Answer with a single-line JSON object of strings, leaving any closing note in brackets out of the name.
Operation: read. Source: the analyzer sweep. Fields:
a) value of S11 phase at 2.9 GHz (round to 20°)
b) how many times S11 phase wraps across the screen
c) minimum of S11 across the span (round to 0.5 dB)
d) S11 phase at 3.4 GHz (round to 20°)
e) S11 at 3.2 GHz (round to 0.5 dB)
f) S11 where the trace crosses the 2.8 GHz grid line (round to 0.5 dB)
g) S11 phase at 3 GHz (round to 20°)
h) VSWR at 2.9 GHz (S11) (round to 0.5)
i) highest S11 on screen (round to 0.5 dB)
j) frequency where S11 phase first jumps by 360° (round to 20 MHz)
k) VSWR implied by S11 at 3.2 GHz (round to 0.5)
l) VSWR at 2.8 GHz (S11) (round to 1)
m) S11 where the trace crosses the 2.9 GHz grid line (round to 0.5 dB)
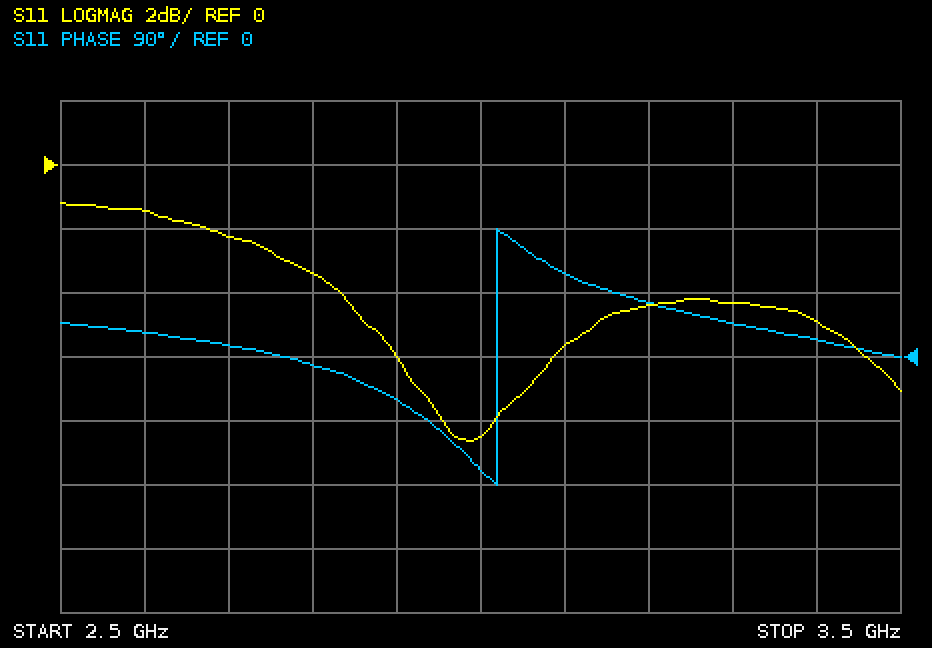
{"value of S11 phase at 2.9 GHz": "-60°", "how many times S11 phase wraps across the screen": "1", "minimum of S11 across the span": "-8.5 dB", "S11 phase at 3.4 GHz": "20°", "S11 at 3.2 GHz": "-4.5 dB", "S11 where the trace crosses the 2.8 GHz grid line": "-3.5 dB", "S11 phase at 3 GHz": "-160°", "VSWR at 2.9 GHz (S11)": "3.0", "highest S11 on screen": "-1.0 dB", "frequency where S11 phase first jumps by 360°": "3.02 GHz", "VSWR implied by S11 at 3.2 GHz": "4.0", "VSWR at 2.8 GHz (S11)": "5", "S11 where the trace crosses the 2.9 GHz grid line": "-6.0 dB"}
